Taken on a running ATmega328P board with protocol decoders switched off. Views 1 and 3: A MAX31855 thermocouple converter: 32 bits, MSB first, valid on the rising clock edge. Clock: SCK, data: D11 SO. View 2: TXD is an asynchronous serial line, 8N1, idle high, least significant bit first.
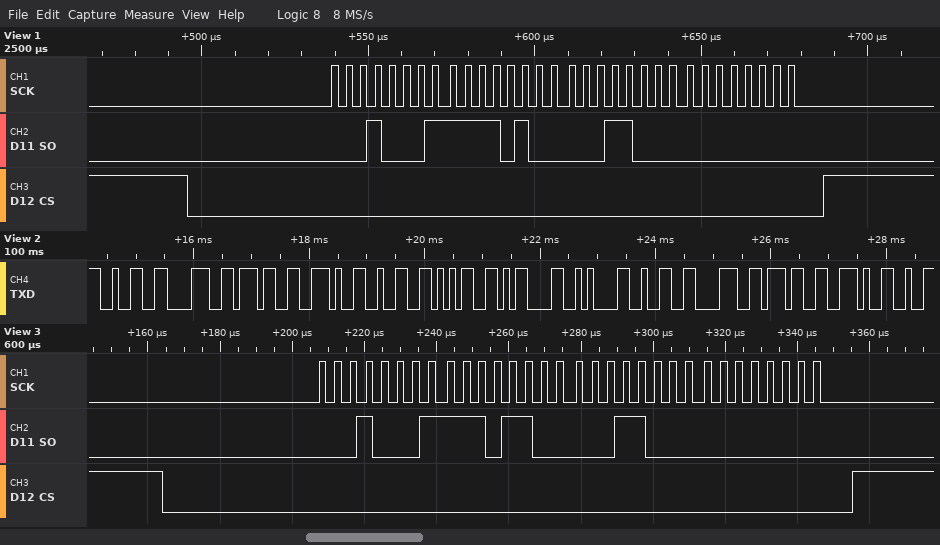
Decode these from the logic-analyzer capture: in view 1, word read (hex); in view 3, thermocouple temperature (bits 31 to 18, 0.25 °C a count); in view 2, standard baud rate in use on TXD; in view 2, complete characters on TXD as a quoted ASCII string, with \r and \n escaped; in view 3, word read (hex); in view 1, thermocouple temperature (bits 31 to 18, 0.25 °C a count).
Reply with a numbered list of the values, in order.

1. 0x11F41800
2. 286.75 °C
3. 9600 baud
4. "287.25\r\n287."
5. 0x11EC1800
6. 287.25 °C
